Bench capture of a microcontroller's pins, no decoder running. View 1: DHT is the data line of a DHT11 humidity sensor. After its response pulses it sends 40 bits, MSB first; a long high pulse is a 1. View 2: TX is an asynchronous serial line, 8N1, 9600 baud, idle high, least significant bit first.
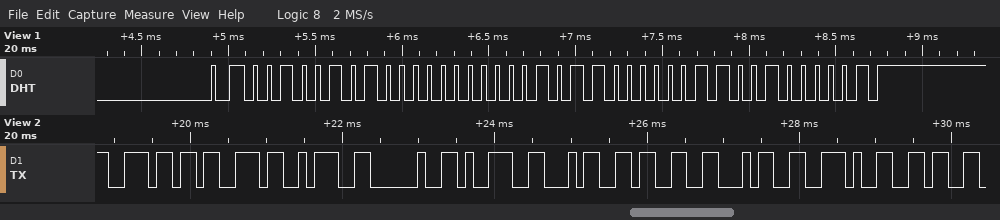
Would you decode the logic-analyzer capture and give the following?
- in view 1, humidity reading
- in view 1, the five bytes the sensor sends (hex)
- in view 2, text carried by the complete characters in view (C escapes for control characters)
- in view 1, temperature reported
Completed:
37 %
25 00 16 06 41
"ns: 9434.6"
22.6 °C
